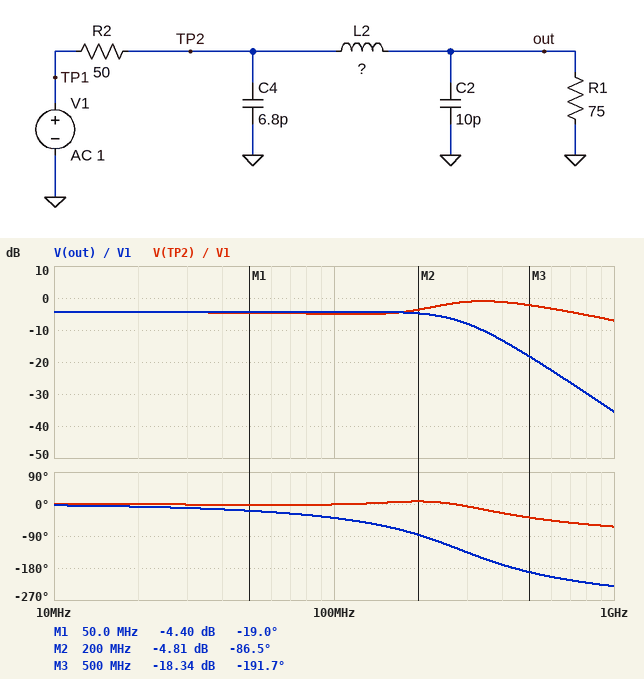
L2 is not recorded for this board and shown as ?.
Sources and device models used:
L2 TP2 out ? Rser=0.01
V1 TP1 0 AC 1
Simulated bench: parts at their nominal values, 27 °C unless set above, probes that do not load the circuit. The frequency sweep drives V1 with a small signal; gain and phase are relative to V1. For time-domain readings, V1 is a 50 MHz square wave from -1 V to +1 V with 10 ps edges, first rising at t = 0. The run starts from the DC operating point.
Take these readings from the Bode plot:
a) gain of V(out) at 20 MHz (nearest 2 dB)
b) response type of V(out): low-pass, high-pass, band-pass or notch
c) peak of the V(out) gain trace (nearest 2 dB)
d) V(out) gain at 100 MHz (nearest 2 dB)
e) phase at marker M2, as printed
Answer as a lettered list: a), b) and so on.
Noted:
a) -4 dB
b) low-pass
c) -4 dB
d) -4 dB
e) -86.5 deg
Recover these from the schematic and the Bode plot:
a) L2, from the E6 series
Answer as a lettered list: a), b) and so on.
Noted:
a) 68 nH
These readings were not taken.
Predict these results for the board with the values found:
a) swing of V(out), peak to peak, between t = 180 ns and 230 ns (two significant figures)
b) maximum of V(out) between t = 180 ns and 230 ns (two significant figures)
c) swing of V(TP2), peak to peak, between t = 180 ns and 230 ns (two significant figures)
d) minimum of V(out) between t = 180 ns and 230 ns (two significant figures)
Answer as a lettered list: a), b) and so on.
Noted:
a) 1.4 V
b) 710 mV
c) 1.8 V
d) -710 mV
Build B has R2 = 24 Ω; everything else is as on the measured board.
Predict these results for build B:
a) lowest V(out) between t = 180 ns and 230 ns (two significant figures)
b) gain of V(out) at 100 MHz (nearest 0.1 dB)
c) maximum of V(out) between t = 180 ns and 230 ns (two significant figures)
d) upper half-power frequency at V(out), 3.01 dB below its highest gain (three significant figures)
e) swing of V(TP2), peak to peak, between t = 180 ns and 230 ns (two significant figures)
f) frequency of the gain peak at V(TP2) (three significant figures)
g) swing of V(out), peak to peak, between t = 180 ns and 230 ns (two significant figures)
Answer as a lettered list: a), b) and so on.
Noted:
a) -910 mV
b) -2.1 dB
c) 910 mV
d) 251 MHz
e) 2.0 V
f) 370 MHz
g) 1.8 V
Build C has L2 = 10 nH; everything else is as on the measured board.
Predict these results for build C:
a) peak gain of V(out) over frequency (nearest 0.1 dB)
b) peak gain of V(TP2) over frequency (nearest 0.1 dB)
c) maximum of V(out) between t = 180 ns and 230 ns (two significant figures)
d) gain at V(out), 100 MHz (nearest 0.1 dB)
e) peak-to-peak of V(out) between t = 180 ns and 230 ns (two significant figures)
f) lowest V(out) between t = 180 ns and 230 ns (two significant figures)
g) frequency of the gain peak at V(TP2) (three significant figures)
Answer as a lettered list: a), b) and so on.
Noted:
a) -4.4 dB
b) -1.9 dB
c) 630 mV
d) -4.7 dB
e) 1.3 V
f) -630 mV
g) 825 MHz
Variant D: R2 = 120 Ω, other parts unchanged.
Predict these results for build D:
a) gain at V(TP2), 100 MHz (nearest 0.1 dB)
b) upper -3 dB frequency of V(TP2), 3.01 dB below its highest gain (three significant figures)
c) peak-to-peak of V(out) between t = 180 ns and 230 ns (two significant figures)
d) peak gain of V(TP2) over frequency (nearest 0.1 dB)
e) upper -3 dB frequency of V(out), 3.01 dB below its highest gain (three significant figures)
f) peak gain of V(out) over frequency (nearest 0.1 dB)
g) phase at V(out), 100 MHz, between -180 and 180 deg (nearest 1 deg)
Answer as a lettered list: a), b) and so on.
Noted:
a) -9.1 dB
b) 452 MHz
c) 930 mV
d) -2.6 dB
e) 329 MHz
f) -8.2 dB
g) -40 deg
